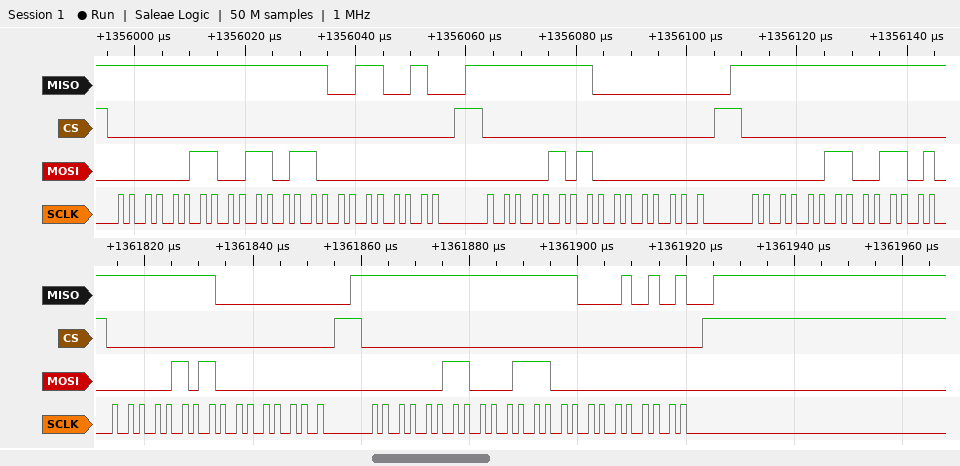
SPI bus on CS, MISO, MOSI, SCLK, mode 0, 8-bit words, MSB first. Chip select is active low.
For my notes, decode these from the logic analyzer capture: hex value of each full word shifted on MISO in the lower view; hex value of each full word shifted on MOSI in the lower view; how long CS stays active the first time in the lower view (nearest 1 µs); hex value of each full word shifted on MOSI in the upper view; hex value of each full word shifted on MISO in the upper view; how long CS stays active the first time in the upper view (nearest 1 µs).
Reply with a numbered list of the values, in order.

1. FF, 00, FF, FF, 15
2. 05, 00, 03, 1C, 00
3. 42 µs
4. 03, 36, 00, 05, 00, 03
5. FF, FF, 32, FF, 00, FF
6. 63 µs
